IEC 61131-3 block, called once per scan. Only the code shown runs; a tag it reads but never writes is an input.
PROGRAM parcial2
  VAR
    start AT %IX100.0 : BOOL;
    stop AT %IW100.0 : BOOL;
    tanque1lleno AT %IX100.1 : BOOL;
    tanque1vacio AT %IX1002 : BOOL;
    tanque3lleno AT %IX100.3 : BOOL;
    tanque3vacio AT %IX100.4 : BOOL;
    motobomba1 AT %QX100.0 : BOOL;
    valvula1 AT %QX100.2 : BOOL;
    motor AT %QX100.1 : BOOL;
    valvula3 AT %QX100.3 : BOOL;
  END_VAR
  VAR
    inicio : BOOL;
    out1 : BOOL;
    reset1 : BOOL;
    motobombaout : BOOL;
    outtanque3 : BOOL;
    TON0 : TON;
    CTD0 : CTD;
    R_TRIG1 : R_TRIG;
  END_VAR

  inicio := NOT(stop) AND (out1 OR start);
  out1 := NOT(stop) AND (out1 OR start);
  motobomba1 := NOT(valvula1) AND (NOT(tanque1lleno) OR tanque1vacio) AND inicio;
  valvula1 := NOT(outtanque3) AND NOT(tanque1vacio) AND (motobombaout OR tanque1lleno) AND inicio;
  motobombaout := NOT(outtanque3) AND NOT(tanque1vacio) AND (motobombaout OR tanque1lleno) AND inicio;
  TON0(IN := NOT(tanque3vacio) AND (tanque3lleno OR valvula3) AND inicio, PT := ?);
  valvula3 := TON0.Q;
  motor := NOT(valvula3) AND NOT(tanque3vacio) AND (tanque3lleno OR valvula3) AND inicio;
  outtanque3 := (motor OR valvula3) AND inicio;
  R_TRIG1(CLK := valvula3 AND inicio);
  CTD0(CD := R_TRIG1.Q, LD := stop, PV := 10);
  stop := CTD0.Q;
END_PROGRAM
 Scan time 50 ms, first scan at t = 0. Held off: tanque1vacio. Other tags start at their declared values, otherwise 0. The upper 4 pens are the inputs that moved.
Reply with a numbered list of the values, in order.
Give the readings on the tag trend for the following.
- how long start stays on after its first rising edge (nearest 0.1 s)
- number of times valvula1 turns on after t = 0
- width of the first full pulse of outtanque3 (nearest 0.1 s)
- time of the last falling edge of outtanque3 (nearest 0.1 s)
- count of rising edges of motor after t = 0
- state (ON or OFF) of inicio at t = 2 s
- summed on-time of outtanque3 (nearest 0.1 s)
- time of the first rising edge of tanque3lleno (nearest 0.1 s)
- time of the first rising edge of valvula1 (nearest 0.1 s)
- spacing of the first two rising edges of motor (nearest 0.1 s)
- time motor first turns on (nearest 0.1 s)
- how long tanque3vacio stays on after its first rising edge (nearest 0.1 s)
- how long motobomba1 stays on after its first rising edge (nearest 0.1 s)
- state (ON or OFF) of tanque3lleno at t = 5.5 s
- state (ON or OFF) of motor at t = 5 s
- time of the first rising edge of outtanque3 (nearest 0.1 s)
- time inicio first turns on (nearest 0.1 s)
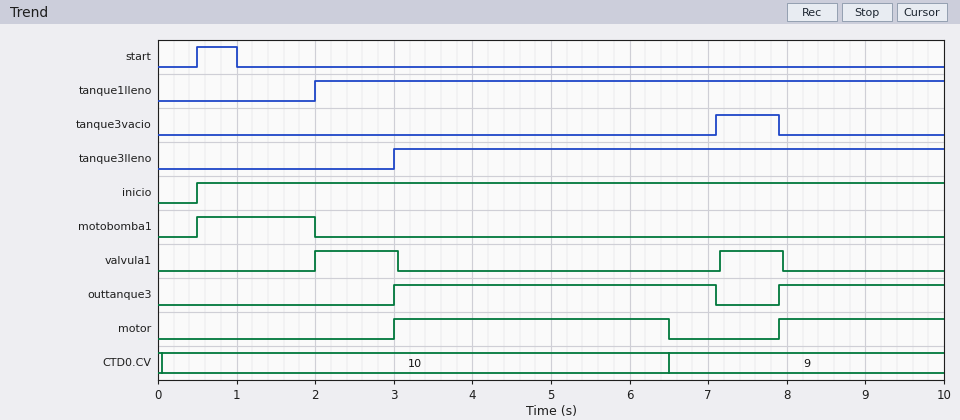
1. 0.5 s
2. 2
3. 4.1 s
4. 7.1 s
5. 2
6. ON
7. 6.2 s
8. 3.0 s
9. 2.0 s
10. 4.9 s
11. 3.0 s
12. 0.8 s
13. 1.5 s
14. ON
15. ON
16. 3.0 s
17. 0.5 s
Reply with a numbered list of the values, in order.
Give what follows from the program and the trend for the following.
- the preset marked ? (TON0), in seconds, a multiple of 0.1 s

1. 3.5 s
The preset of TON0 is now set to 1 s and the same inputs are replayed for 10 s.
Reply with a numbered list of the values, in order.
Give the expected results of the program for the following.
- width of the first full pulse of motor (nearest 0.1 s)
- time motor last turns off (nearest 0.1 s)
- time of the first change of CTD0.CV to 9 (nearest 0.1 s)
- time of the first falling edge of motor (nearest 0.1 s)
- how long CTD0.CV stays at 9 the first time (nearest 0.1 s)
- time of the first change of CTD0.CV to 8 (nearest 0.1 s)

1. 1.0 s
2. 8.9 s
3. 4.0 s
4. 4.0 s
5. 4.9 s
6. 8.9 s
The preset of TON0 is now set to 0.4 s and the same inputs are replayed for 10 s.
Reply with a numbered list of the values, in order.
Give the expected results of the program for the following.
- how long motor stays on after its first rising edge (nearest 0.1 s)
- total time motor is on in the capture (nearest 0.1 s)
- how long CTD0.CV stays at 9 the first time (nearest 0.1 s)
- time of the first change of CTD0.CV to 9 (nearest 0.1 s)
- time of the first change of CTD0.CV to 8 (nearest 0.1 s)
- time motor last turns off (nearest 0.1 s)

1. 0.4 s
2. 0.8 s
3. 4.9 s
4. 3.4 s
5. 8.3 s
6. 8.3 s
